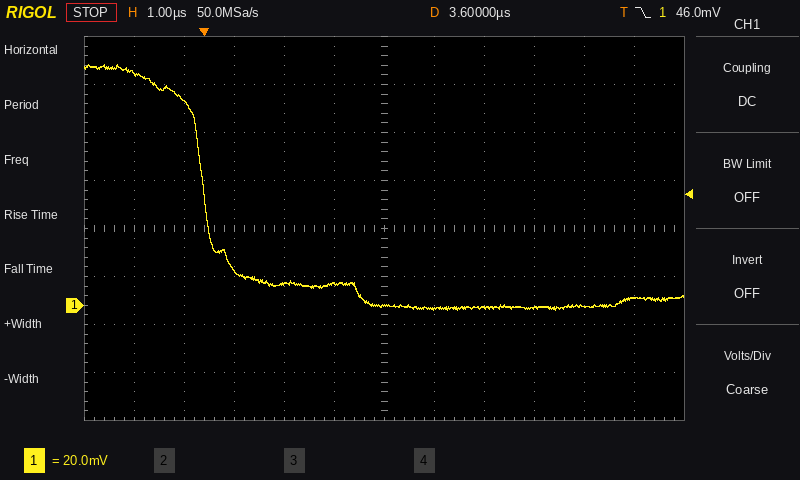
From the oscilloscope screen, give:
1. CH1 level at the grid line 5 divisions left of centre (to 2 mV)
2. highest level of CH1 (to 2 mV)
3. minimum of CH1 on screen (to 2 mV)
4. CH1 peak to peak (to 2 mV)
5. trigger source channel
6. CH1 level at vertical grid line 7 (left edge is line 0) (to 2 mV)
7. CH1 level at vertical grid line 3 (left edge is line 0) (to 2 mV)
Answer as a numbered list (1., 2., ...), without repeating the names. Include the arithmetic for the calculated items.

1. 96 mV
2. 100 mV
3. -2 mV
4. 100 mV − (-2 mV) = 102 mV
5. CH1
6. -2 mV
7. 14 mV
